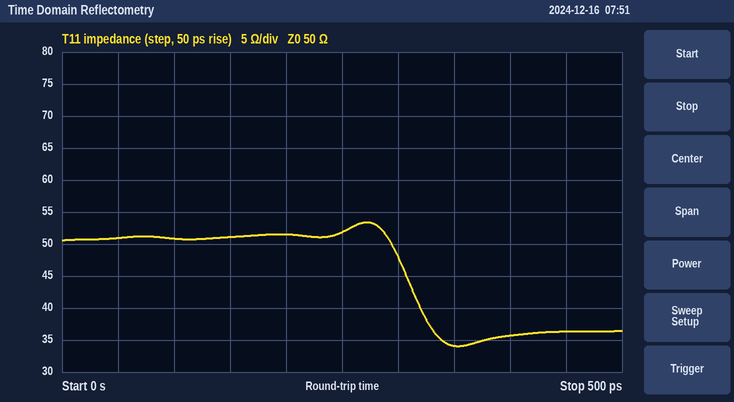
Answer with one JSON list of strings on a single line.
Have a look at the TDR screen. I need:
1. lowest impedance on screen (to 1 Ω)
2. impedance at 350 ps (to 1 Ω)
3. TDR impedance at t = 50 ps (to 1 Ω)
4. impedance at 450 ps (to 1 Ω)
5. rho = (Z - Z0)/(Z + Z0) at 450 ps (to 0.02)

["34 Ω", "34 Ω", "51 Ω", "36 Ω", "-0.16"]
